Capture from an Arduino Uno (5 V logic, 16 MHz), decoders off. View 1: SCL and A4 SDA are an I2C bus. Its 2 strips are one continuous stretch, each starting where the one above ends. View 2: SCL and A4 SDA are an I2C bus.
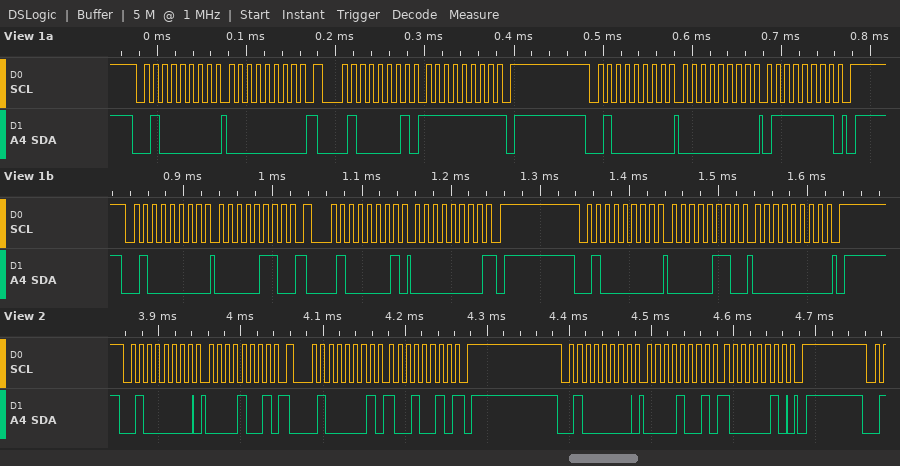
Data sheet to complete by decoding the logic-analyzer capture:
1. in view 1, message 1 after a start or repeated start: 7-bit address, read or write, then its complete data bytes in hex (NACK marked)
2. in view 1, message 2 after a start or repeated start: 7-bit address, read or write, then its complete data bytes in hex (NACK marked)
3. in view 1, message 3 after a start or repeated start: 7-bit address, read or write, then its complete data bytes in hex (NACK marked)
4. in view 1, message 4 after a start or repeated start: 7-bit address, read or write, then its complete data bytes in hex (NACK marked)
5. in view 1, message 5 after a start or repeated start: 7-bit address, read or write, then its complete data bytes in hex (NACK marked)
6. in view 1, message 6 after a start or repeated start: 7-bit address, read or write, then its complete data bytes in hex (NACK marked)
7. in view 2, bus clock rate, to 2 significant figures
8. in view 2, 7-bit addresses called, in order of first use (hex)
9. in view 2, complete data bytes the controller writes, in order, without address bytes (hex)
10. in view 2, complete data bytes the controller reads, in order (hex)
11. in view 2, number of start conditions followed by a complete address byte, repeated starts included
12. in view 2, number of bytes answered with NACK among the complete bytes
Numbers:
0x20 write: 00
0x20 read: FF NACK
0x20 write: 00 7F
0x20 write: 06
0x20 read: 00 NACK
0x20 write: 06 00
100 kHz
0x20
09 09 82
92
3
1
